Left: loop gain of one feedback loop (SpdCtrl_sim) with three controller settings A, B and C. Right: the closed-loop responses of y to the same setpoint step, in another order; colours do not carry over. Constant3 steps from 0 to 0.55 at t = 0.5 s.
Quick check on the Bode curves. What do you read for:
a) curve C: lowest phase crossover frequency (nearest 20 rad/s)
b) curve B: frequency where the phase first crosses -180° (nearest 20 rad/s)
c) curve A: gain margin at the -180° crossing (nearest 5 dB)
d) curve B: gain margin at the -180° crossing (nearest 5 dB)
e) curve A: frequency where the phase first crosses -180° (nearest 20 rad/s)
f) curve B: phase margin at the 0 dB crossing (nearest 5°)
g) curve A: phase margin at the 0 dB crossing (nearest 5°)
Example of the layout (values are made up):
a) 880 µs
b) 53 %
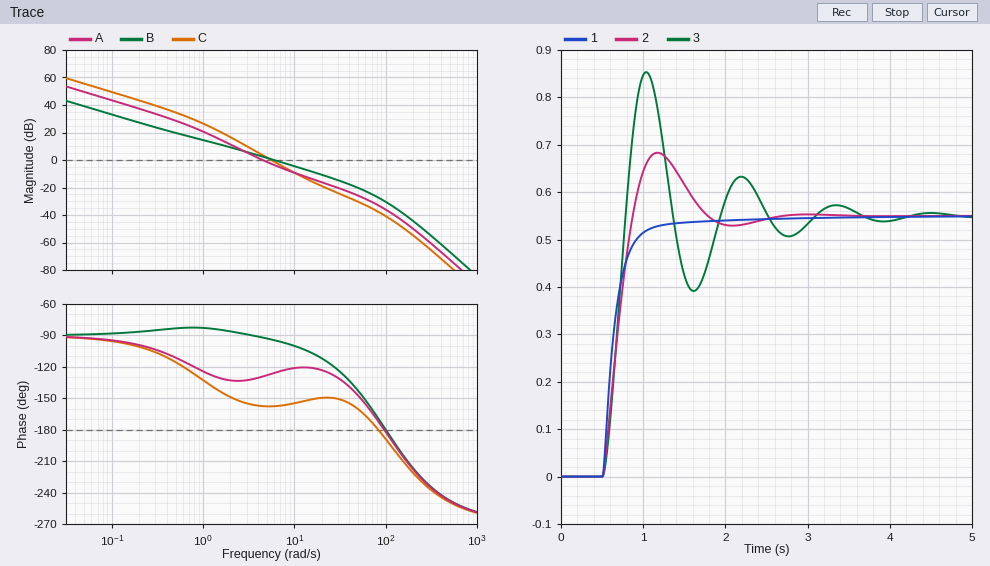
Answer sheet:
a) 80 rad/s
b) 100 rad/s
c) 35 dB
d) 30 dB
e) 100 rad/s
f) 85°
g) 50°
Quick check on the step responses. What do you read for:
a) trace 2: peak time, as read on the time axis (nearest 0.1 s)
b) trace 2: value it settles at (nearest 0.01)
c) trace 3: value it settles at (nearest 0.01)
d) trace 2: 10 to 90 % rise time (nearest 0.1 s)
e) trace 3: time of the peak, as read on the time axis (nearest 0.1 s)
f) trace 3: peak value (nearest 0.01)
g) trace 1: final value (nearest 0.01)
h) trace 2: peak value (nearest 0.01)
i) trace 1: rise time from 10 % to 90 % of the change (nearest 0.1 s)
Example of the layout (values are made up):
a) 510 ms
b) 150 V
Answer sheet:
a) 1.2 s
b) 0.55
c) 0.55
d) 0.3 s
e) 1.0 s
f) 0.85
g) 0.55
h) 0.68
i) 0.4 s
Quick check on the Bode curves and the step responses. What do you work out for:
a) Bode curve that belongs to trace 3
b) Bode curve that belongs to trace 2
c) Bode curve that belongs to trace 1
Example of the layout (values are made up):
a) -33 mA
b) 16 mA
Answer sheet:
a) C
b) A
c) B
